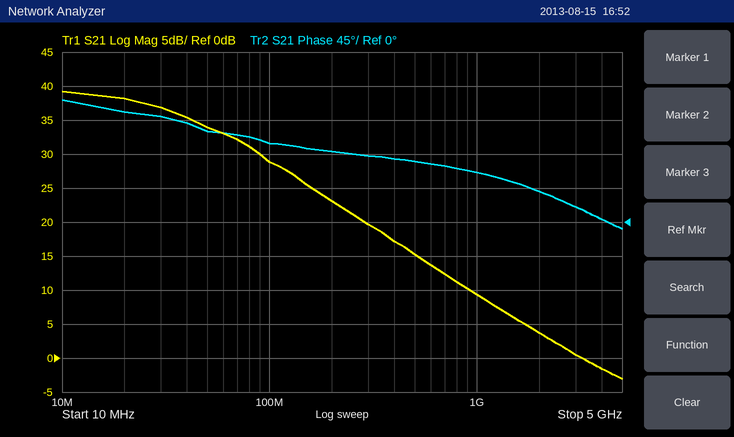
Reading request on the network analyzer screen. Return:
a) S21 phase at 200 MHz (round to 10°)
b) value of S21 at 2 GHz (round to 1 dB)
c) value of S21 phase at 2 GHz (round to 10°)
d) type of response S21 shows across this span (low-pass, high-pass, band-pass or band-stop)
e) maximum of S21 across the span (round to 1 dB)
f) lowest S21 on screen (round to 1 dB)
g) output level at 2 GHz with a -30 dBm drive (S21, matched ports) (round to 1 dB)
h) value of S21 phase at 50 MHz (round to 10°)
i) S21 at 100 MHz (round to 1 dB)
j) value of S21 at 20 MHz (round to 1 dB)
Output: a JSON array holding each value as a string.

["90°", "4 dB", "40°", "low-pass", "39 dB", "-3 dB", "-26 dBm", "120°", "29 dB", "38 dB"]
